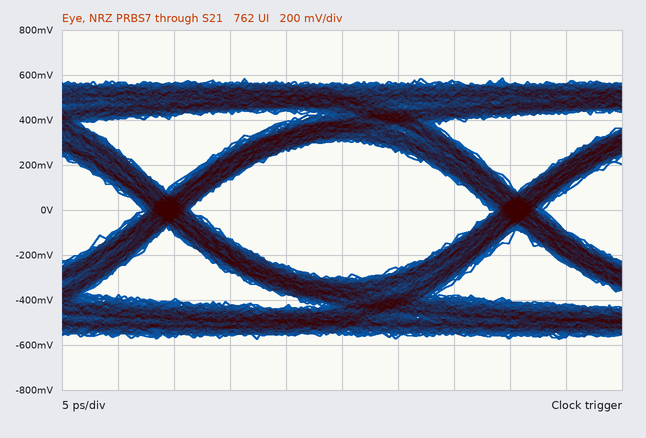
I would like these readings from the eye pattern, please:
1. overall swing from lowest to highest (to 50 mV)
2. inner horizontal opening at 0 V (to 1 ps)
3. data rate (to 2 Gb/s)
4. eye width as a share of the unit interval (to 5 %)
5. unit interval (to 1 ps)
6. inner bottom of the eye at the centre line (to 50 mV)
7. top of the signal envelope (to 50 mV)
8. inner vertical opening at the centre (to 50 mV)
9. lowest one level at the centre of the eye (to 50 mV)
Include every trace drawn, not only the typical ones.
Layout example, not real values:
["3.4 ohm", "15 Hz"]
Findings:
["1.15 V", "27 ps", "32 Gb/s", "85 %", "31 ps", "-300 mV", "600 mV", "600 mV", "300 mV"]
